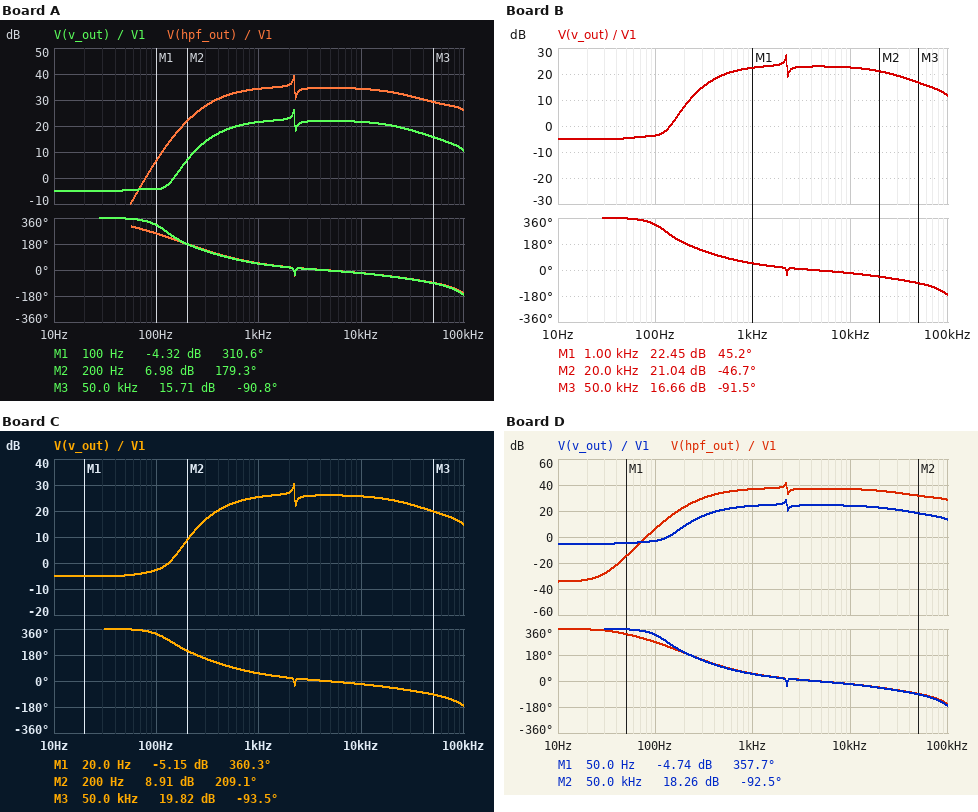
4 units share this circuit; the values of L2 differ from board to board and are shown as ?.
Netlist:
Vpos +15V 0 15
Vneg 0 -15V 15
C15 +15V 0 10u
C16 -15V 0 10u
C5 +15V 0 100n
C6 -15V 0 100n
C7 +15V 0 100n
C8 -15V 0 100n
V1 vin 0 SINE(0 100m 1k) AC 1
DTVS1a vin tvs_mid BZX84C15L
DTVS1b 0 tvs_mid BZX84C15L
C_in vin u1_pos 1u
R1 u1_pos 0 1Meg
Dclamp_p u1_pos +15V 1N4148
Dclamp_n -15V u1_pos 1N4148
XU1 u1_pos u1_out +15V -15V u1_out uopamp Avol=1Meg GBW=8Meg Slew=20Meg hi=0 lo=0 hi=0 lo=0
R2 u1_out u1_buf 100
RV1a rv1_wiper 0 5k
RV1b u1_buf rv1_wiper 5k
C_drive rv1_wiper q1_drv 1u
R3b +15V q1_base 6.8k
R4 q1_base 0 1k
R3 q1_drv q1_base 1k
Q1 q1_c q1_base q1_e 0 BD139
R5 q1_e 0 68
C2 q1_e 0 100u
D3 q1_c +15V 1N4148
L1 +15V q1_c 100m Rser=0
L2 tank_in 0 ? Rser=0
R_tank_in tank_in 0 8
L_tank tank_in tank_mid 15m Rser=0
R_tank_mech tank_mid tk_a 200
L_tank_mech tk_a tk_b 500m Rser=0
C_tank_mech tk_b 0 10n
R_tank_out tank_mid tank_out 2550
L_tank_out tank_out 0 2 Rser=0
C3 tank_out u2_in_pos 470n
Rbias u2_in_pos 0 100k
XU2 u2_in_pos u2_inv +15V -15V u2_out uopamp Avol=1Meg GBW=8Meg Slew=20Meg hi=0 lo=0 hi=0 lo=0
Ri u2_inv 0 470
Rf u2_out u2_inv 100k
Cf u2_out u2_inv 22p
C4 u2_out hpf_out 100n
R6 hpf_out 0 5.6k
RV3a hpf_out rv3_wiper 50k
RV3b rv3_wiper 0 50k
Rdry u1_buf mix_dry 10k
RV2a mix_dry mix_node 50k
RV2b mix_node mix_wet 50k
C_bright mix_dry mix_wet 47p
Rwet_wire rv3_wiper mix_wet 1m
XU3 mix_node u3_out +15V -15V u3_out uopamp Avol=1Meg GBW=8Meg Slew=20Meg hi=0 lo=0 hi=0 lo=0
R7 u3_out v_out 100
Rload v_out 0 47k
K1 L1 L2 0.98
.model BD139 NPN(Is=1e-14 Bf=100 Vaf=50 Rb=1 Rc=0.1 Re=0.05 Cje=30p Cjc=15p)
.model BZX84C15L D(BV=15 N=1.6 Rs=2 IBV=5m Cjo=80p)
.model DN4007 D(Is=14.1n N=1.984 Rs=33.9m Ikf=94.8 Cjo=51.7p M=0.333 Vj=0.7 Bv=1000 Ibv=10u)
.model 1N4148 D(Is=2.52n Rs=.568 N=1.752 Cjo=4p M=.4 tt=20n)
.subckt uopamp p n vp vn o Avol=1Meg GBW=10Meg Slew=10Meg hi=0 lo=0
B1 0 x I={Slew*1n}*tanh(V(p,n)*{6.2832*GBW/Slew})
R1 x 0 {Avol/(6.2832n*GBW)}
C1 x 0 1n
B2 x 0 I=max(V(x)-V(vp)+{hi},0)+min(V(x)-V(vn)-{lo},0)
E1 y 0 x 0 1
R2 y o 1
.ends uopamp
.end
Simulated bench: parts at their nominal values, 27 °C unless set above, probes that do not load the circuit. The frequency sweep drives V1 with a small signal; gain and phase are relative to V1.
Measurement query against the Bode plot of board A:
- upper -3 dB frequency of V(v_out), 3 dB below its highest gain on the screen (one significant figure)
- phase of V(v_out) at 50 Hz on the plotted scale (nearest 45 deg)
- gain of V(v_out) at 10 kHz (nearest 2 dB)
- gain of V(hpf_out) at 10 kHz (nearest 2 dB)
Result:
2 kHz
360 deg
22 dB
34 dB
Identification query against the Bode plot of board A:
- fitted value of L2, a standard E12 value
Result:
15 mH
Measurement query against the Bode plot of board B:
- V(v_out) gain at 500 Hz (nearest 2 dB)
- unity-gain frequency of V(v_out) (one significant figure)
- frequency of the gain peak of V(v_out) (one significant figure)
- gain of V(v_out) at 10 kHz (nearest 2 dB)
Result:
20 dB
100 Hz
2 kHz
22 dB
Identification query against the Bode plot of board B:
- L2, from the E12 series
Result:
12 mH
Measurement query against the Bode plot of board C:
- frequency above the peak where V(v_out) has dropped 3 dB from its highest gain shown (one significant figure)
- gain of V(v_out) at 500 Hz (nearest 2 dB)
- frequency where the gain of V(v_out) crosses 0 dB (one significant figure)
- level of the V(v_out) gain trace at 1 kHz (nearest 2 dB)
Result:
2 kHz
22 dB
100 Hz
26 dB
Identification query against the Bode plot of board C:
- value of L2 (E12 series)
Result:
5.6 mH
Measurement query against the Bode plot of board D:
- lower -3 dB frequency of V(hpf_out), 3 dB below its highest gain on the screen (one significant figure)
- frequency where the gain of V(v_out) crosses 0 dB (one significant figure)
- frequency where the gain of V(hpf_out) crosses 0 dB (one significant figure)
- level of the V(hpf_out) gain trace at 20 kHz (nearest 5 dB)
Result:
2 kHz
100 Hz
80 Hz
35 dB
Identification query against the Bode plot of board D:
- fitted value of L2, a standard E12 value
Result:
8.2 mH
